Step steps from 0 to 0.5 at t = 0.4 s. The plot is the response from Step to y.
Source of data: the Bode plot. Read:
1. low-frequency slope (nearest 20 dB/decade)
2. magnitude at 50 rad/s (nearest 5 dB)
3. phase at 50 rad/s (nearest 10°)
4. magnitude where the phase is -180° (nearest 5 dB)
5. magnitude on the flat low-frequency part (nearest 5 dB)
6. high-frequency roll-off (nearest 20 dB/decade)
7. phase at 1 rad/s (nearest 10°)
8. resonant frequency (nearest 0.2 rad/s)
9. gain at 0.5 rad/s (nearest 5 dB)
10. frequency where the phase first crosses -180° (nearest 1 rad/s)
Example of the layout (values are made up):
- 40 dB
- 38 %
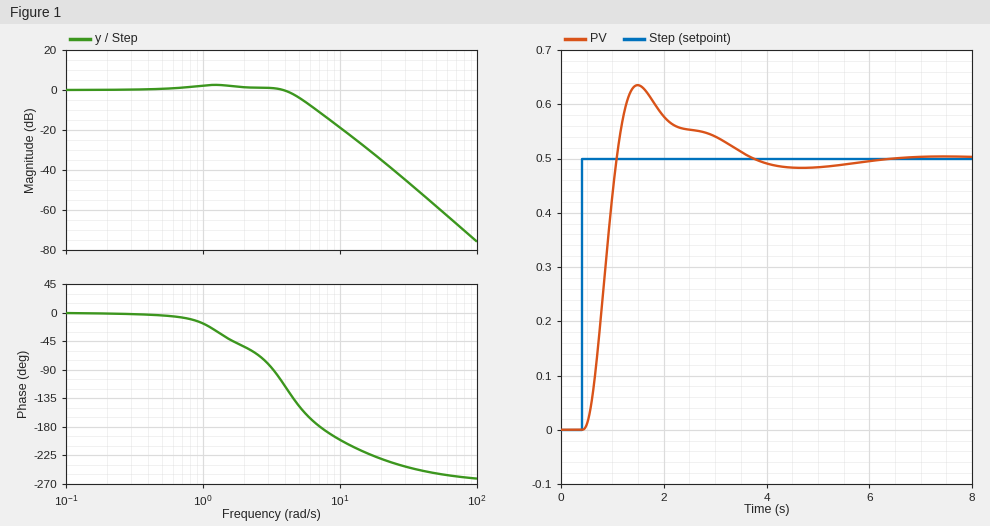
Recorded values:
- 0 dB/decade
- -60 dB
- -250°
- -10 dB
- 0 dB
- -60 dB/decade
- -20°
- 1.2 rad/s
- 0 dB
- 7 rad/s
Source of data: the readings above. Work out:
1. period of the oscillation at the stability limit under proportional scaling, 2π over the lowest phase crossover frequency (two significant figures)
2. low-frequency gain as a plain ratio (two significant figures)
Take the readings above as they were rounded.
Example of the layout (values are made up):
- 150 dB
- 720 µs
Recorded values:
- 0.90 s
- 1.0
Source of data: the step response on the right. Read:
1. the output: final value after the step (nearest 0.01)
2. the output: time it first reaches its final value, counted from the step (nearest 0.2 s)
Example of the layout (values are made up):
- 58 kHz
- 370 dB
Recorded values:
- 0.50
- 0.6 s
